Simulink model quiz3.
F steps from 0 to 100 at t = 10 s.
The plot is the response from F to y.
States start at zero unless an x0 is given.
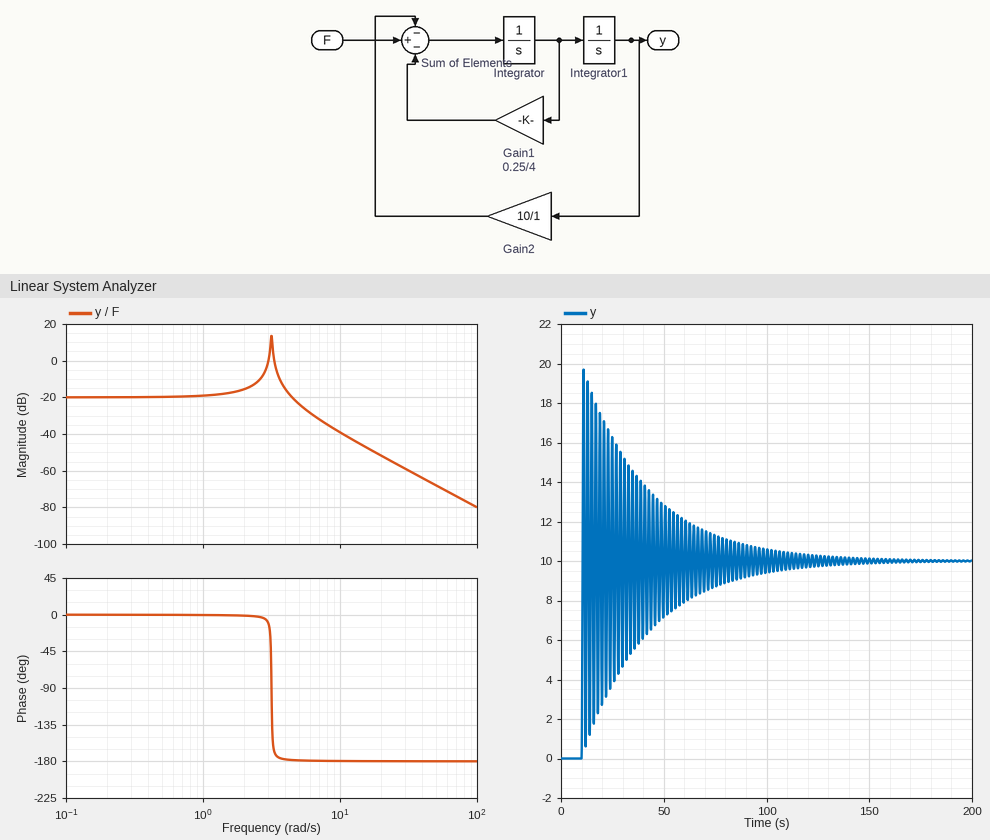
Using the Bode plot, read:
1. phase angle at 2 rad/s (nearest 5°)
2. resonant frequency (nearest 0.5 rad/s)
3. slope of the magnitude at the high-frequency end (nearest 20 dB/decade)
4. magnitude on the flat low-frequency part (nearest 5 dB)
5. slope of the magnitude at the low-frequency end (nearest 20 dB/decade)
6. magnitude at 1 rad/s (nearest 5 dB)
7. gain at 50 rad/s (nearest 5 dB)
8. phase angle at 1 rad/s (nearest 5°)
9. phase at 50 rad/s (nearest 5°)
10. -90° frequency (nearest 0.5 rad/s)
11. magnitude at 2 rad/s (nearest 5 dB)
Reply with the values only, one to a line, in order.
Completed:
0°
3.0 rad/s
-40 dB/decade
-20 dB
0 dB/decade
-20 dB
-70 dB
0°
-180°
3.0 rad/s
-15 dB
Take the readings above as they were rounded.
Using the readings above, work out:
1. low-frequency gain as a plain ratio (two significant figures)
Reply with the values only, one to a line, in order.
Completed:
0.10
